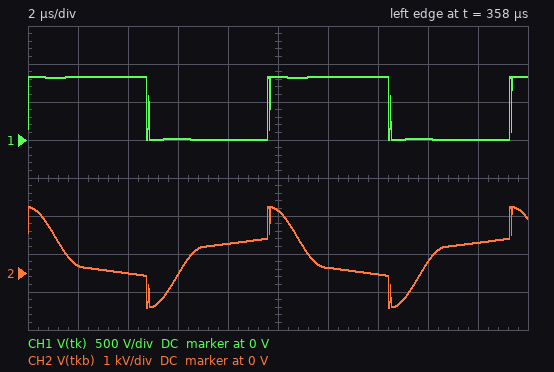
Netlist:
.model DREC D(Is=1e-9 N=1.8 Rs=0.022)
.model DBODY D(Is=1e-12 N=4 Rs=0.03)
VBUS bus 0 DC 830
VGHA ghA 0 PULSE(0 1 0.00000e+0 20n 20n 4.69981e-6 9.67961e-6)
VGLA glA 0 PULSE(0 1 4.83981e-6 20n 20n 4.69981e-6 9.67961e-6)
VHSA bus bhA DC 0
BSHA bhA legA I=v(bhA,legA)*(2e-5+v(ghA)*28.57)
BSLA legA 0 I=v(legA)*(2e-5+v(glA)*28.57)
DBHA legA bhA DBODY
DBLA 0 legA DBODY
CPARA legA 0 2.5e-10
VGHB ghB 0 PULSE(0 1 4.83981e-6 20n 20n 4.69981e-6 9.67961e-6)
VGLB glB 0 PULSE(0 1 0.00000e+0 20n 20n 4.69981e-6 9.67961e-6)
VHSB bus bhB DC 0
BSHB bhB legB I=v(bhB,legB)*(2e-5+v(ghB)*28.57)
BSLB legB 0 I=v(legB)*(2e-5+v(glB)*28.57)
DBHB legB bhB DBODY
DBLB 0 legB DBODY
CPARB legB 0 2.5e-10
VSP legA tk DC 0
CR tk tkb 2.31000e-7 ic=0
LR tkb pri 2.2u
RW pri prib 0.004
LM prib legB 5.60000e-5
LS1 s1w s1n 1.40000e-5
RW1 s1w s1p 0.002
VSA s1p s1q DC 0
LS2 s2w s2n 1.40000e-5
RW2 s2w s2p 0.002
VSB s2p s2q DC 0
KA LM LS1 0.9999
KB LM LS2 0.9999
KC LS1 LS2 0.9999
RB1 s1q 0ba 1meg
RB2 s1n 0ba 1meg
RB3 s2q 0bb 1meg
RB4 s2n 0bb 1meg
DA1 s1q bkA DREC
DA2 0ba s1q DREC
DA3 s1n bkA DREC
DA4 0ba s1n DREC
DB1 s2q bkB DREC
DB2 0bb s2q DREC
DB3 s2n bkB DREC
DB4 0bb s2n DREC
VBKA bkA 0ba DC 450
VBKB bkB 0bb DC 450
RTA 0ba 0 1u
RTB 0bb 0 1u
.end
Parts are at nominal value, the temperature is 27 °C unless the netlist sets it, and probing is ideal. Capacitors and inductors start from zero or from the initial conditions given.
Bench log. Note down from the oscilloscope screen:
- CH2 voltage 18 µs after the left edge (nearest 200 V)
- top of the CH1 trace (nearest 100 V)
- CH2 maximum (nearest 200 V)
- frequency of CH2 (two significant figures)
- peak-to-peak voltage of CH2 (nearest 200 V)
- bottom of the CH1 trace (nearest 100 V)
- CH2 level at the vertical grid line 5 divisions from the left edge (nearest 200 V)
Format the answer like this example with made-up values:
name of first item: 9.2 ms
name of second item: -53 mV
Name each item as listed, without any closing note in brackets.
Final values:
CH2 voltage 18 µs after the left edge: 800 V
top of the CH1 trace: 800 V
CH2 maximum: 1.8 kV
frequency of CH2: 100 kHz
peak-to-peak voltage of CH2: 2.6 kV
bottom of the CH1 trace: 0 V
CH2 level at the vertical grid line 5 divisions from the left edge: 1.6 kV
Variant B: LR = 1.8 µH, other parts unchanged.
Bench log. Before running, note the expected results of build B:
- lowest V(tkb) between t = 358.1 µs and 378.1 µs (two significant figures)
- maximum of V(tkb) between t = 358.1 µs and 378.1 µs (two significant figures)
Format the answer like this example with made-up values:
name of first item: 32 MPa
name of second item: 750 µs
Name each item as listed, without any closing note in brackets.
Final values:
lowest V(tkb) between t = 358.1 µs and 378.1 µs: -820 V
maximum of V(tkb) between t = 358.1 µs and 378.1 µs: 1.6 kV
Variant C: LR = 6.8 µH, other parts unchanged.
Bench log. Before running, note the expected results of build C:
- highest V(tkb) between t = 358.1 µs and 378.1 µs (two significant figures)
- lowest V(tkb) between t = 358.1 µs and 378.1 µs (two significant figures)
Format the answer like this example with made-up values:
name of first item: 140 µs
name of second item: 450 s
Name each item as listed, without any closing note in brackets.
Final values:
highest V(tkb) between t = 358.1 µs and 378.1 µs: 1.0 kV
lowest V(tkb) between t = 358.1 µs and 378.1 µs: -210 V
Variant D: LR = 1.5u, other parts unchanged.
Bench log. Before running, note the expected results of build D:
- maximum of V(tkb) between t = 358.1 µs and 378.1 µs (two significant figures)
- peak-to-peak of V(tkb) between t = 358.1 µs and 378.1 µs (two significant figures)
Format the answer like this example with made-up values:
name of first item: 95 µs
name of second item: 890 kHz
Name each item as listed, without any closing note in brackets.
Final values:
maximum of V(tkb) between t = 358.1 µs and 378.1 µs: 1.5 kV
peak-to-peak of V(tkb) between t = 358.1 µs and 378.1 µs: 2.3 kV
